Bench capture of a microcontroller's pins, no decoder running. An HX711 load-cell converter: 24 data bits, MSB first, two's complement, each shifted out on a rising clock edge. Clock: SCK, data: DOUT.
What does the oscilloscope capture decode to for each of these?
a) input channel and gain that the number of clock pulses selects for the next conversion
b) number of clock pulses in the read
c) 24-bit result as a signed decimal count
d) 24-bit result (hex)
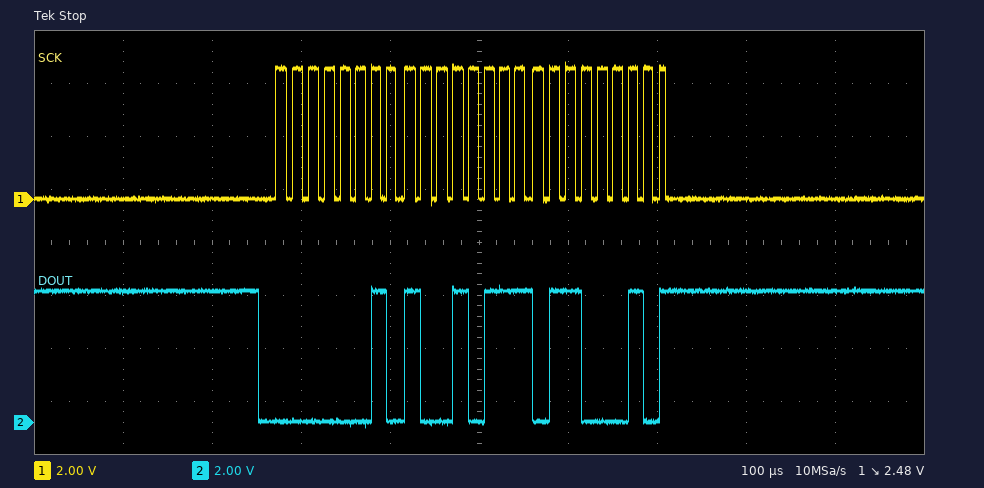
channel A, gain 128
25
169826
0x029762
